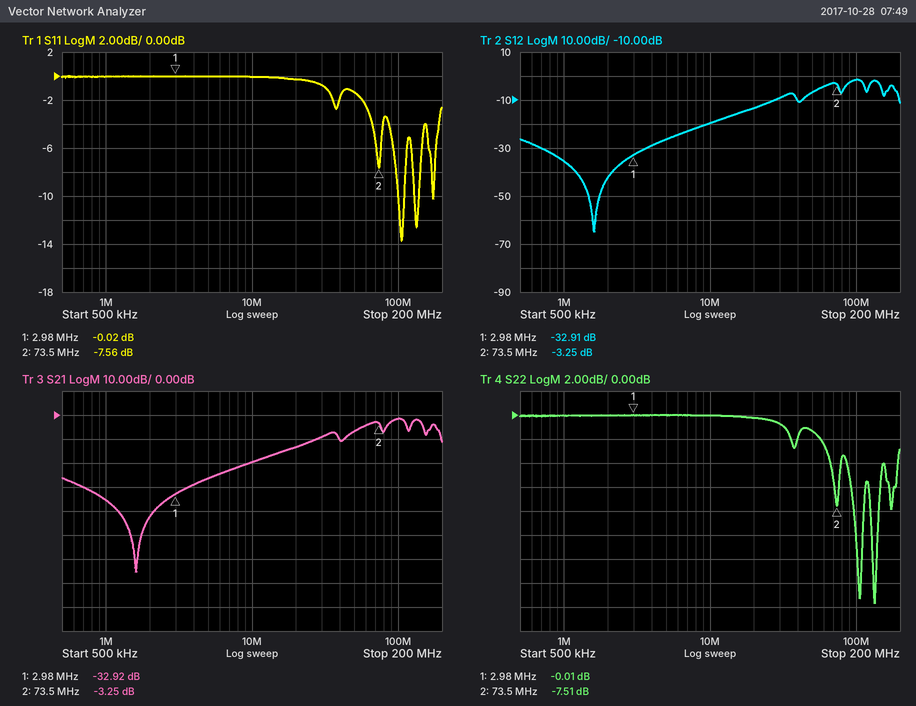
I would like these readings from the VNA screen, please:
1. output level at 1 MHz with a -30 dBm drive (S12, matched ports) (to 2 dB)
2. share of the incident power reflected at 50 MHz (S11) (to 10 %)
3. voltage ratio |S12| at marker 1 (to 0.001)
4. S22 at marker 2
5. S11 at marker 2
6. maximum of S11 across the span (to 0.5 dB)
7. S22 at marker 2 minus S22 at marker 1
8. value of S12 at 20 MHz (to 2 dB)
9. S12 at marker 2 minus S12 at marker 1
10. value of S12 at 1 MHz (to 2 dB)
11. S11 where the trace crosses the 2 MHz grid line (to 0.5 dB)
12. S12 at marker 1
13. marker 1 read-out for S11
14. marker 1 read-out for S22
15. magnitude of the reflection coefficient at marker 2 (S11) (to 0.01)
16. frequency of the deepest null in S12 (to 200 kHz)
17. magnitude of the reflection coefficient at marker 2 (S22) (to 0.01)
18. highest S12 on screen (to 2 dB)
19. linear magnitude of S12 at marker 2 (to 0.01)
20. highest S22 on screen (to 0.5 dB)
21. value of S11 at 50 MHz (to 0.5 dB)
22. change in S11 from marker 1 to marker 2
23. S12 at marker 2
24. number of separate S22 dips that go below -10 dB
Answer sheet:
-66 dBm
70 %
0.023
-7.51 dB
-7.56 dB
0.0 dB
-7.50 dB
-14 dB
29.66 dB
-36 dB
0.0 dB
-32.91 dB
-0.02 dB
-0.01 dB
0.42
1.6 MHz
0.42
-2 dB
0.69
0.0 dB
-1.5 dB
-7.54 dB
-3.25 dB
2
